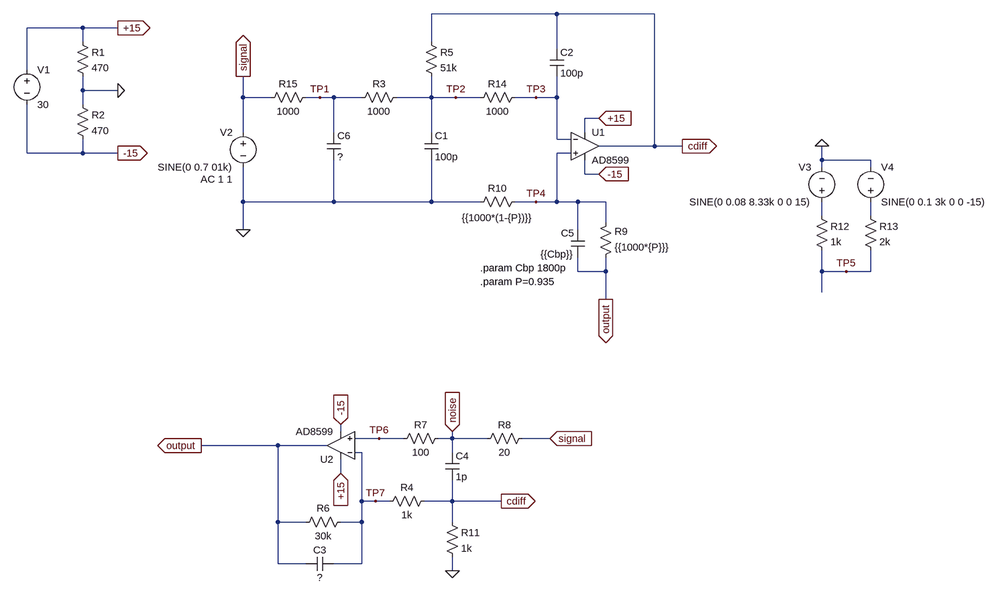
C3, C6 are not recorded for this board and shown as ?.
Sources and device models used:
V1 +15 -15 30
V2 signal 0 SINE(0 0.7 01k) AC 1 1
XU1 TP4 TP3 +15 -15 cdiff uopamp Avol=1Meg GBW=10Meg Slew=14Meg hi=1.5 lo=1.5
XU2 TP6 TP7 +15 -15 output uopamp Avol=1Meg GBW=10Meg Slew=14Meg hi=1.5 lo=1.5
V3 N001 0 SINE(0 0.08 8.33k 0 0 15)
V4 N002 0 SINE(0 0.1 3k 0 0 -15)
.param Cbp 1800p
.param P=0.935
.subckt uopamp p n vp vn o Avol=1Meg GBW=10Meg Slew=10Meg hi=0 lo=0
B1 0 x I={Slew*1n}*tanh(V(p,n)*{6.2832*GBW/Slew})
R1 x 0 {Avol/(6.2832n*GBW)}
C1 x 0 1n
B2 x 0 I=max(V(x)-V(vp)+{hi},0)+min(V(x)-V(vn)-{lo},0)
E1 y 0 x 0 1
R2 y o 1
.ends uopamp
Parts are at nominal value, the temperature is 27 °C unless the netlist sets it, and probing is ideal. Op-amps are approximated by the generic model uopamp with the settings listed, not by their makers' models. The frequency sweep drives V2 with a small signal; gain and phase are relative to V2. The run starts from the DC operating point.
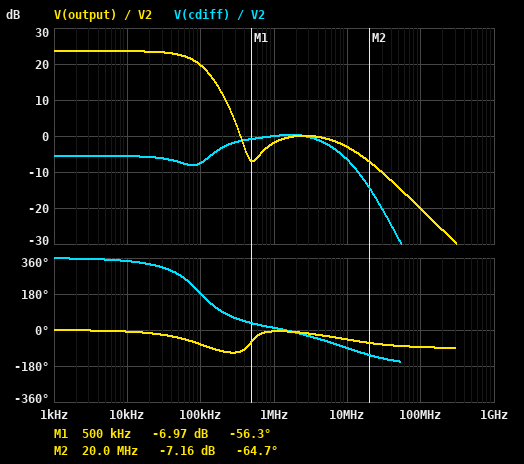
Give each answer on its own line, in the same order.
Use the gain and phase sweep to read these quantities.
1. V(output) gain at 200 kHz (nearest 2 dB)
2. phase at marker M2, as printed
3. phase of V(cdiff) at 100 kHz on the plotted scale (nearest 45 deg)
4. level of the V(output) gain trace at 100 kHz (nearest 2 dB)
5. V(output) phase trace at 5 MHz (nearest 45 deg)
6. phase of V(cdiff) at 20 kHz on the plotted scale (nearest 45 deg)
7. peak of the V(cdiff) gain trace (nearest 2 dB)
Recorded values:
12 dB
-64.7 deg
180 deg
20 dB
-45 deg
315 deg
0 dB
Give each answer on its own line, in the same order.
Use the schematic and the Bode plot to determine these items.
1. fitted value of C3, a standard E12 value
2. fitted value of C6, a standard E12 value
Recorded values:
220 pF
220 pF
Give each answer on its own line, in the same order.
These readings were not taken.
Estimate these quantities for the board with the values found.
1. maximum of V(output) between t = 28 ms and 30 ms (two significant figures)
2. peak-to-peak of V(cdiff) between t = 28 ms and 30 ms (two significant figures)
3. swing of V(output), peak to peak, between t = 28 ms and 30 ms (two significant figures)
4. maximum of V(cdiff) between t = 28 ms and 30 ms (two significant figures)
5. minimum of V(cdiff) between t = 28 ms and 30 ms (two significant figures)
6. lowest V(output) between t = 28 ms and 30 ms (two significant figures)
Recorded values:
11 V
740 mV
21 V
370 mV
-370 mV
-11 V
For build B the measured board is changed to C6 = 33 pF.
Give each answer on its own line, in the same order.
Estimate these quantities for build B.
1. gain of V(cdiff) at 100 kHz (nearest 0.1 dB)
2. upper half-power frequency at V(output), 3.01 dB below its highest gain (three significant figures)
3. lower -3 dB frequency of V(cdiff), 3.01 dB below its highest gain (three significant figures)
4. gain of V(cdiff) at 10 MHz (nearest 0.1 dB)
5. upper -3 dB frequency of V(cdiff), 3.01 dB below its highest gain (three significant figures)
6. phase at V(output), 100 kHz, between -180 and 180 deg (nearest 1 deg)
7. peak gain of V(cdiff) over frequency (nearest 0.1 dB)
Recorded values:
-6.1 dB
91.9 kHz
471 kHz
-6.5 dB
5.60 MHz
-66 deg
0.6 dB
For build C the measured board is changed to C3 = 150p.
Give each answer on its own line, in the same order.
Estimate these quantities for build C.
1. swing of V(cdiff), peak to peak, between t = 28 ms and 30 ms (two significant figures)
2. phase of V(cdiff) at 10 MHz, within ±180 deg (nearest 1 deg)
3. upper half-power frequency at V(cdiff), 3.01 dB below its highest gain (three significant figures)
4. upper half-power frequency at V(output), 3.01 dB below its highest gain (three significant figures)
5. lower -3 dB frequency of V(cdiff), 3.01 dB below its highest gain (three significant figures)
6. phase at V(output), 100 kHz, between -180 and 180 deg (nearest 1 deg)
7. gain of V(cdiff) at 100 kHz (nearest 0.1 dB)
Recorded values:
740 mV
-91 deg
5.85 MHz
85.8 kHz
335 kHz
-67 deg
-36.2 dB
